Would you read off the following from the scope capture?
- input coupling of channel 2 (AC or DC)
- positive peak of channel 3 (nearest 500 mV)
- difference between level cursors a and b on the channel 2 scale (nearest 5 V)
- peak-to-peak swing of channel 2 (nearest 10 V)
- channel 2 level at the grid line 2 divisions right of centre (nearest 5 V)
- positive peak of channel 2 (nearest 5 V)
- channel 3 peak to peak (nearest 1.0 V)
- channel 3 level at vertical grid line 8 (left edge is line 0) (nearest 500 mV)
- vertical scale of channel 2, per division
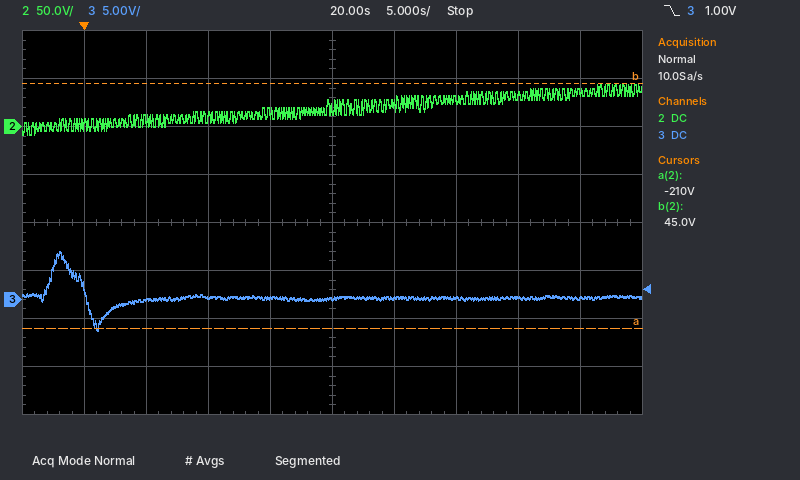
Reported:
DC
5.0 V
255 V
50 V
30 V
45 V
8.0 V
0.0 V
50 V
